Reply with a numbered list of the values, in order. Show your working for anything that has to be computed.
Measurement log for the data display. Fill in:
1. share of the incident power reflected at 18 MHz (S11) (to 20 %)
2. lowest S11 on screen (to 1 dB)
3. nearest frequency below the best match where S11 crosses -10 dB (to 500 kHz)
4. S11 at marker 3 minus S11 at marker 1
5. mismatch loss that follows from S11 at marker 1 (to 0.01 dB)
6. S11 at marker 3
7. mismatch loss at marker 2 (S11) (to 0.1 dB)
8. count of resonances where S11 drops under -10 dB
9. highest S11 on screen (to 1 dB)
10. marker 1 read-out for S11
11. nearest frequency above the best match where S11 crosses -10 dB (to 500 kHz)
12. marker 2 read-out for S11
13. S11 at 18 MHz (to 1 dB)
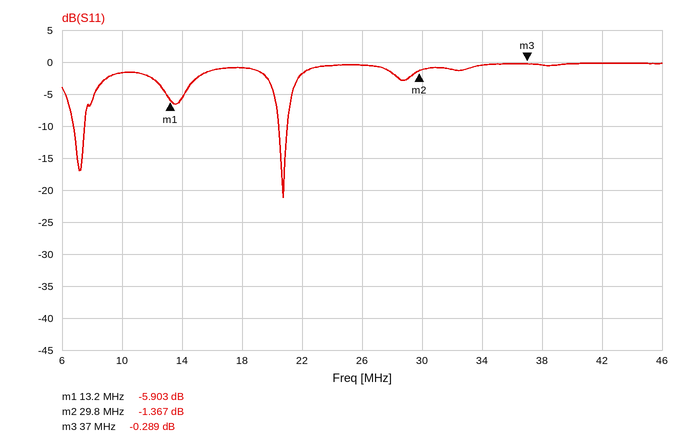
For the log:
1. 10^(-1/10) ≈ 79.4 %, so 80 % to the nearest 20 %
2. -21 dB
3. 20.5 MHz
4. -0.289 − (-5.903) = 5.614 dB
5. −10 log10(1 − 10^(-5.903/10)) ≈ 1.29 dB
6. -0.289 dB
7. −10 log10(1 − 10^(-1.367/10)) ≈ 5.7 dB
8. 2
9. 0 dB
10. -5.903 dB
11. 21.0 MHz
12. -1.367 dB
13. -1 dB
